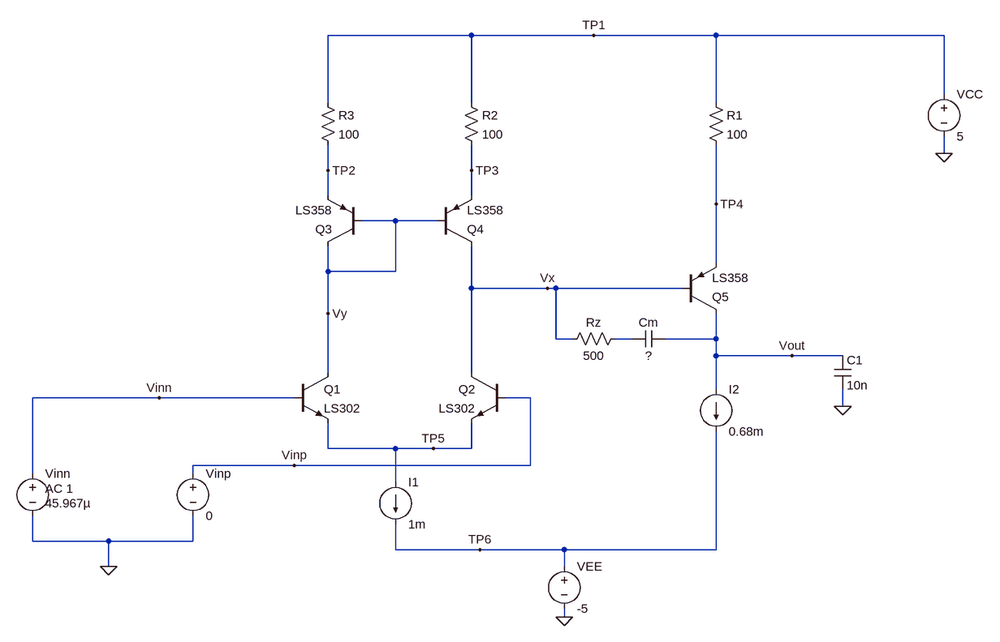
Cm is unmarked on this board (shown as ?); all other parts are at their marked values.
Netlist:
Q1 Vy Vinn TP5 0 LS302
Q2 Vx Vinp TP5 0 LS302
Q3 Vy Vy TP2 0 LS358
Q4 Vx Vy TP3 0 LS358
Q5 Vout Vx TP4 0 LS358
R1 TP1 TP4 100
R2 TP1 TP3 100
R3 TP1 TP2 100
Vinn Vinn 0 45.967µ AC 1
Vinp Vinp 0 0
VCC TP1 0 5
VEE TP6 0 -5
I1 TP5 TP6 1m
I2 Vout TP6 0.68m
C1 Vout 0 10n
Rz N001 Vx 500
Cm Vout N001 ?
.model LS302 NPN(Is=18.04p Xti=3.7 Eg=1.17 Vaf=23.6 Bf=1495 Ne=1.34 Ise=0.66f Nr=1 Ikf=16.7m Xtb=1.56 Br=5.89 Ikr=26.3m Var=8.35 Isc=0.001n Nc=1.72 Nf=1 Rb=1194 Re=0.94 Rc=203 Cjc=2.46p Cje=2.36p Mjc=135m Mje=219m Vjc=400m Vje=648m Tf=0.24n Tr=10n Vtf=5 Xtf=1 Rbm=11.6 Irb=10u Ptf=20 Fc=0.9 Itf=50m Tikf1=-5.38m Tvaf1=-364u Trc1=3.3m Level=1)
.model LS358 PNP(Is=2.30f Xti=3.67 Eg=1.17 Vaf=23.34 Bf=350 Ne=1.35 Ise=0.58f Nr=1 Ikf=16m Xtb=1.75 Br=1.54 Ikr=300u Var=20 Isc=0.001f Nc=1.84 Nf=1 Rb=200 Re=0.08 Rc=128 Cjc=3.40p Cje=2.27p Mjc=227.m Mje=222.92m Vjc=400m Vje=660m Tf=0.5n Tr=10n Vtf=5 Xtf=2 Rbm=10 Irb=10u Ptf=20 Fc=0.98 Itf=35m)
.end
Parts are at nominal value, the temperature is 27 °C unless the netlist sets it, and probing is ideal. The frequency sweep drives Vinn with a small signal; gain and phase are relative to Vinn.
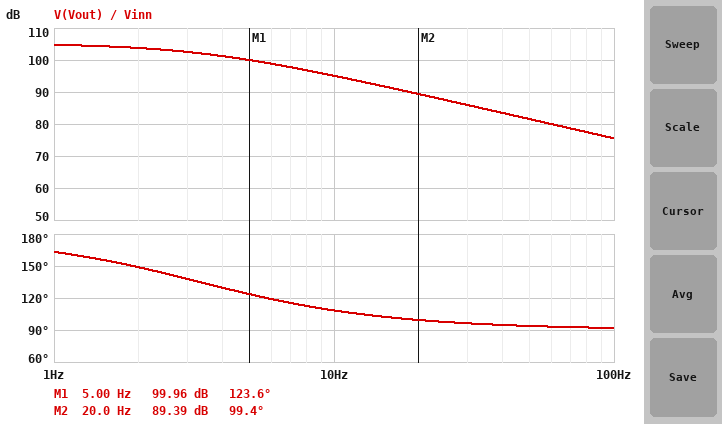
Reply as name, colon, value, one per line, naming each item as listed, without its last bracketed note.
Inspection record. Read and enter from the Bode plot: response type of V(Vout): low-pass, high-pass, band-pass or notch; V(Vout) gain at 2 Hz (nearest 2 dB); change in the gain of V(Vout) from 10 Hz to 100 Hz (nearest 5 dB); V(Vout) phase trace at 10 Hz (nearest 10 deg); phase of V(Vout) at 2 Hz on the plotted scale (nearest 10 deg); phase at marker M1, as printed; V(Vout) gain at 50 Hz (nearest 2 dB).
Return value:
response type of V(Vout): low-pass, high-pass, band-pass or notch: low-pass
V(Vout) gain at 2 Hz: 104 dB
change in the gain of V(Vout) from 10 Hz to 100 Hz: -20 dB
V(Vout) phase trace at 10 Hz: 110 deg
phase of V(Vout) at 2 Hz on the plotted scale: 150 deg
phase at marker M1, as printed: 123.6 deg
V(Vout) gain at 50 Hz: 82 dB
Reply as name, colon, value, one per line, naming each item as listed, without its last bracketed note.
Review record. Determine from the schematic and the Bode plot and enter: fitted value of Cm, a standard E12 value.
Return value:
fitted value of Cm, a standard E12 value: 4.7 nF
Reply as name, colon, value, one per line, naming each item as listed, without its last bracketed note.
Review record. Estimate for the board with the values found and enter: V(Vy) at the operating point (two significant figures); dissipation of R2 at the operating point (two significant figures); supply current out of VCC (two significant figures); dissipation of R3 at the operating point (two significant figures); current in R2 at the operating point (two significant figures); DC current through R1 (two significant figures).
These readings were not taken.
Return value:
V(Vy) at the operating point: 4.3 V
dissipation of R2 at the operating point: 25 µW
supply current out of VCC: 1.7 mA
dissipation of R3 at the operating point: 25 µW
current in R2 at the operating point: 500 µA
DC current through R1: 680 µA
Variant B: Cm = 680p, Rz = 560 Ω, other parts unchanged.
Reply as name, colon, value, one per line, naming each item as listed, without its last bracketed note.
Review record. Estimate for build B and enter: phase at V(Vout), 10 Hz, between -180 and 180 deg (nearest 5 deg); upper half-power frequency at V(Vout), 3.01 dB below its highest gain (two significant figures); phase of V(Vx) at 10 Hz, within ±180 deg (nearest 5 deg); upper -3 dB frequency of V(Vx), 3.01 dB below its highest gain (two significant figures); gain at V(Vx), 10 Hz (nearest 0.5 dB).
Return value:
phase at V(Vout), 10 Hz, between -180 and 180 deg: 155 deg
upper half-power frequency at V(Vout), 3.01 dB below its highest gain: 21 Hz
phase of V(Vx) at 10 Hz, within ±180 deg: -20 deg
upper -3 dB frequency of V(Vx), 3.01 dB below its highest gain: 22 Hz
gain at V(Vx), 10 Hz: 44.5 dB
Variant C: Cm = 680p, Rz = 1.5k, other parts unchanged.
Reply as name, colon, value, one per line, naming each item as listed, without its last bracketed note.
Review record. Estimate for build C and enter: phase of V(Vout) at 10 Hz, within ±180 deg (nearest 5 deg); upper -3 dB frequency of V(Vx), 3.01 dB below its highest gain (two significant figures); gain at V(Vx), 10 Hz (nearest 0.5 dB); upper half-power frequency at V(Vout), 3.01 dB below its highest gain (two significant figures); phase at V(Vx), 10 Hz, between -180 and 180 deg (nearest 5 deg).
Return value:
phase of V(Vout) at 10 Hz, within ±180 deg: 155 deg
upper -3 dB frequency of V(Vx), 3.01 dB below its highest gain: 22 Hz
gain at V(Vx), 10 Hz: 44.5 dB
upper half-power frequency at V(Vout), 3.01 dB below its highest gain: 21 Hz
phase at V(Vx), 10 Hz, between -180 and 180 deg: -20 deg
